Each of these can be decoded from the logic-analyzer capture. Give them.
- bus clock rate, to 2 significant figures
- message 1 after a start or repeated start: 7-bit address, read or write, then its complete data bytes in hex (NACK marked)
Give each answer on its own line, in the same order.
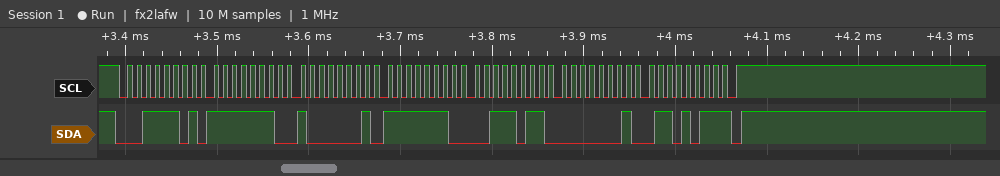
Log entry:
100 kHz
0x1E read: FE 81 FE 3B 01 6B NACK
